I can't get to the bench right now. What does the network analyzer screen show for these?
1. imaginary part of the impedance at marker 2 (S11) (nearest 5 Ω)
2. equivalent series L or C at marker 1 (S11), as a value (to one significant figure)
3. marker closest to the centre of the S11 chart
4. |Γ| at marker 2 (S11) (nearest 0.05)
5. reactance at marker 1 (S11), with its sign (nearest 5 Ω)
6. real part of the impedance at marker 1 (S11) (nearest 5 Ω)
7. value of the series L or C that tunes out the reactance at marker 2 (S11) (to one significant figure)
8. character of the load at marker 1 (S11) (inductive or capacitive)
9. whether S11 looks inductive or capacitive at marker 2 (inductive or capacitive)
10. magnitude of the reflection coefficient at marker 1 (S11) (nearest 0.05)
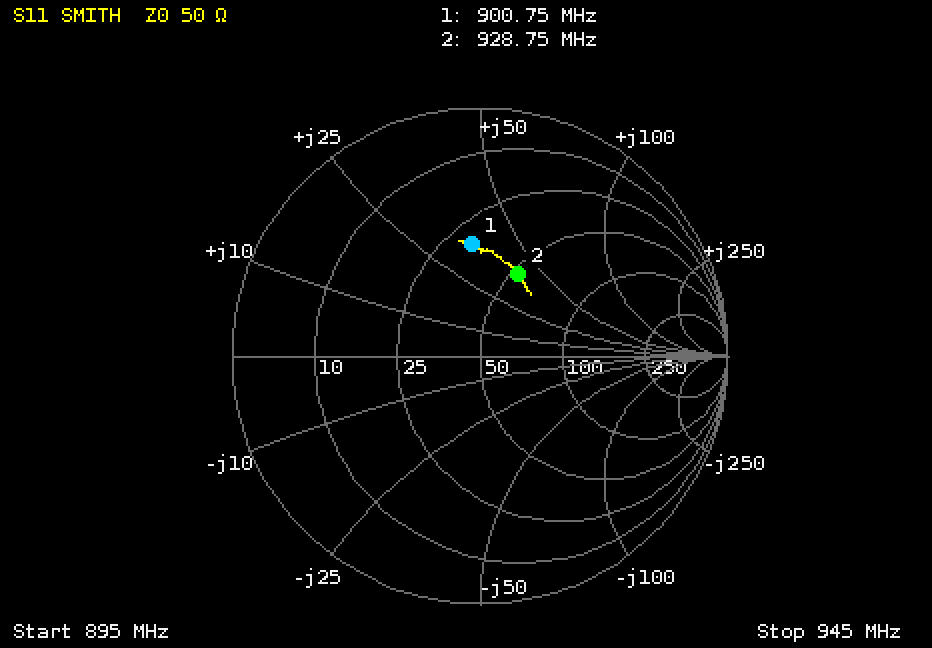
+40 Ω
6 nH
marker 2
0.35
+35 Ω
30 Ω
4 pF
inductive
inductive
0.45
